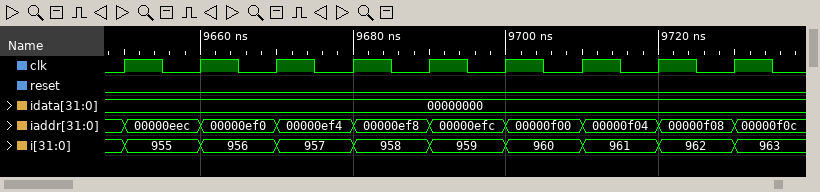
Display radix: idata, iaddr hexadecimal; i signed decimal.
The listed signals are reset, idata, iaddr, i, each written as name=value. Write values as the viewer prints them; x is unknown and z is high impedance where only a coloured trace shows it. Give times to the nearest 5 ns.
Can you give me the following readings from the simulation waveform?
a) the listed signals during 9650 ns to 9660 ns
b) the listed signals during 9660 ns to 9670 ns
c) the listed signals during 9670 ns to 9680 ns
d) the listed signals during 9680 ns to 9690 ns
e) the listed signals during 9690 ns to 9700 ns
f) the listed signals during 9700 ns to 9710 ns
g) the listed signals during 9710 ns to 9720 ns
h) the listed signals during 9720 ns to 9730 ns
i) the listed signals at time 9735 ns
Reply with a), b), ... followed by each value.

a) reset=0, idata=00000000, iaddr=00000eec, i=955
b) reset=0, idata=00000000, iaddr=00000ef0, i=956
c) reset=0, idata=00000000, iaddr=00000ef4, i=957
d) reset=0, idata=00000000, iaddr=00000ef8, i=958
e) reset=0, idata=00000000, iaddr=00000efc, i=959
f) reset=0, idata=00000000, iaddr=00000f00, i=960
g) reset=0, idata=00000000, iaddr=00000f04, i=961
h) reset=0, idata=00000000, iaddr=00000f08, i=962
i) reset=0, idata=00000000, iaddr=00000f0c, i=963
